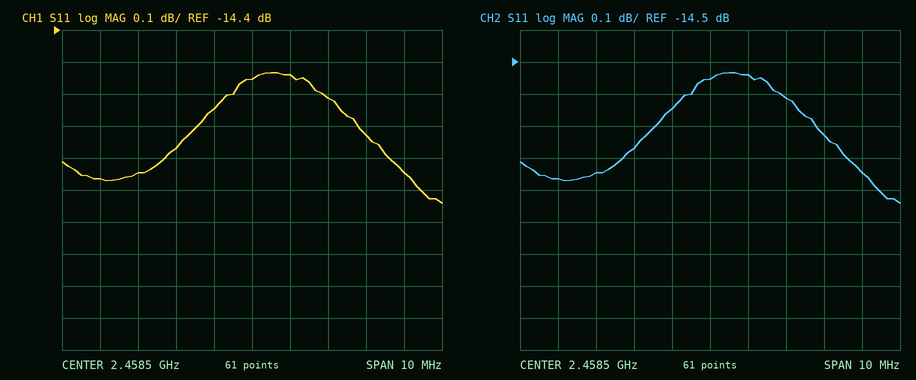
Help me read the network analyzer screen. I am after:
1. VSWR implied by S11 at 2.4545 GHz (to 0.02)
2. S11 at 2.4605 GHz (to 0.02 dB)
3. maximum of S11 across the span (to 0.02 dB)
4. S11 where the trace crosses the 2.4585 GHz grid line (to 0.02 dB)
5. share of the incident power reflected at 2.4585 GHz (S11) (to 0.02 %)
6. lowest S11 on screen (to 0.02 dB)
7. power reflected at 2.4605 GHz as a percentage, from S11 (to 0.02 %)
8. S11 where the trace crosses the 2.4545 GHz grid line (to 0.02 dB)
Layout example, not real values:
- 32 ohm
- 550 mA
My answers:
- 1.44
- -14.62 dB
- -14.54 dB
- -14.56 dB
- 3.50 %
- -14.94 dB
- 3.46 %
- -14.86 dB
